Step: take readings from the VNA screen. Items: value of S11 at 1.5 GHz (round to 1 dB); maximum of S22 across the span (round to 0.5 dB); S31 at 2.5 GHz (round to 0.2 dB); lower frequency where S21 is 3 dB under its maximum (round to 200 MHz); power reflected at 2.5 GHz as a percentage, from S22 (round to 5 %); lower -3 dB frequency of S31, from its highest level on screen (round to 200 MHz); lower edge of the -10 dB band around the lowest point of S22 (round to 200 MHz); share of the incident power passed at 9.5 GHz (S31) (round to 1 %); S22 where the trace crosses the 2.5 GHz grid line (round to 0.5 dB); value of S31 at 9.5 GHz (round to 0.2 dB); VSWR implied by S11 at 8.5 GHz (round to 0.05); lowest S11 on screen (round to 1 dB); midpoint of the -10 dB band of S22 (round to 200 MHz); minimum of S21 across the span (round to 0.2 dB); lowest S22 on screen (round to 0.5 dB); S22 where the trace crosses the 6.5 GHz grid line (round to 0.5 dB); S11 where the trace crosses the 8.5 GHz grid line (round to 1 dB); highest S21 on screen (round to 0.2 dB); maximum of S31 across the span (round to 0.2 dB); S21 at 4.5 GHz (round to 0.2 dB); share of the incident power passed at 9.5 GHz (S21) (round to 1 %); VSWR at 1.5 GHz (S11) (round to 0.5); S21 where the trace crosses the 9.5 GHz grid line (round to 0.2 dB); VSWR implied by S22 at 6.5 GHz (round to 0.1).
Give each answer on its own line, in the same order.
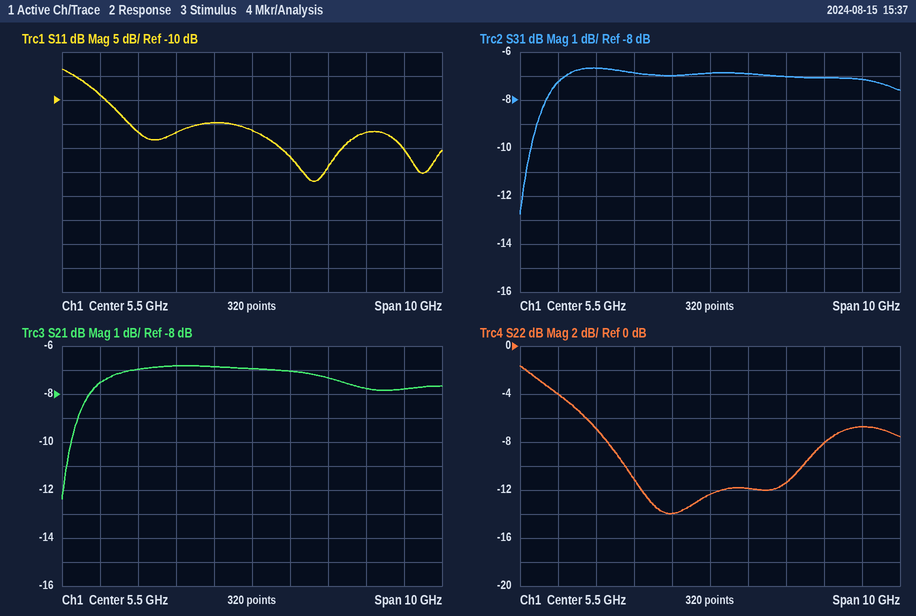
-9 dB
-1.5 dB
-6.6 dB
800 MHz
20 %
800 MHz
3.2 GHz
19 %
-7.0 dB
-7.2 dB
1.35
-27 dB
5.6 GHz
-12.4 dB
-14.0 dB
-12.0 dB
-17 dB
-6.8 dB
-6.6 dB
-6.8 dB
17 %
2.0
-7.8 dB
1.7
